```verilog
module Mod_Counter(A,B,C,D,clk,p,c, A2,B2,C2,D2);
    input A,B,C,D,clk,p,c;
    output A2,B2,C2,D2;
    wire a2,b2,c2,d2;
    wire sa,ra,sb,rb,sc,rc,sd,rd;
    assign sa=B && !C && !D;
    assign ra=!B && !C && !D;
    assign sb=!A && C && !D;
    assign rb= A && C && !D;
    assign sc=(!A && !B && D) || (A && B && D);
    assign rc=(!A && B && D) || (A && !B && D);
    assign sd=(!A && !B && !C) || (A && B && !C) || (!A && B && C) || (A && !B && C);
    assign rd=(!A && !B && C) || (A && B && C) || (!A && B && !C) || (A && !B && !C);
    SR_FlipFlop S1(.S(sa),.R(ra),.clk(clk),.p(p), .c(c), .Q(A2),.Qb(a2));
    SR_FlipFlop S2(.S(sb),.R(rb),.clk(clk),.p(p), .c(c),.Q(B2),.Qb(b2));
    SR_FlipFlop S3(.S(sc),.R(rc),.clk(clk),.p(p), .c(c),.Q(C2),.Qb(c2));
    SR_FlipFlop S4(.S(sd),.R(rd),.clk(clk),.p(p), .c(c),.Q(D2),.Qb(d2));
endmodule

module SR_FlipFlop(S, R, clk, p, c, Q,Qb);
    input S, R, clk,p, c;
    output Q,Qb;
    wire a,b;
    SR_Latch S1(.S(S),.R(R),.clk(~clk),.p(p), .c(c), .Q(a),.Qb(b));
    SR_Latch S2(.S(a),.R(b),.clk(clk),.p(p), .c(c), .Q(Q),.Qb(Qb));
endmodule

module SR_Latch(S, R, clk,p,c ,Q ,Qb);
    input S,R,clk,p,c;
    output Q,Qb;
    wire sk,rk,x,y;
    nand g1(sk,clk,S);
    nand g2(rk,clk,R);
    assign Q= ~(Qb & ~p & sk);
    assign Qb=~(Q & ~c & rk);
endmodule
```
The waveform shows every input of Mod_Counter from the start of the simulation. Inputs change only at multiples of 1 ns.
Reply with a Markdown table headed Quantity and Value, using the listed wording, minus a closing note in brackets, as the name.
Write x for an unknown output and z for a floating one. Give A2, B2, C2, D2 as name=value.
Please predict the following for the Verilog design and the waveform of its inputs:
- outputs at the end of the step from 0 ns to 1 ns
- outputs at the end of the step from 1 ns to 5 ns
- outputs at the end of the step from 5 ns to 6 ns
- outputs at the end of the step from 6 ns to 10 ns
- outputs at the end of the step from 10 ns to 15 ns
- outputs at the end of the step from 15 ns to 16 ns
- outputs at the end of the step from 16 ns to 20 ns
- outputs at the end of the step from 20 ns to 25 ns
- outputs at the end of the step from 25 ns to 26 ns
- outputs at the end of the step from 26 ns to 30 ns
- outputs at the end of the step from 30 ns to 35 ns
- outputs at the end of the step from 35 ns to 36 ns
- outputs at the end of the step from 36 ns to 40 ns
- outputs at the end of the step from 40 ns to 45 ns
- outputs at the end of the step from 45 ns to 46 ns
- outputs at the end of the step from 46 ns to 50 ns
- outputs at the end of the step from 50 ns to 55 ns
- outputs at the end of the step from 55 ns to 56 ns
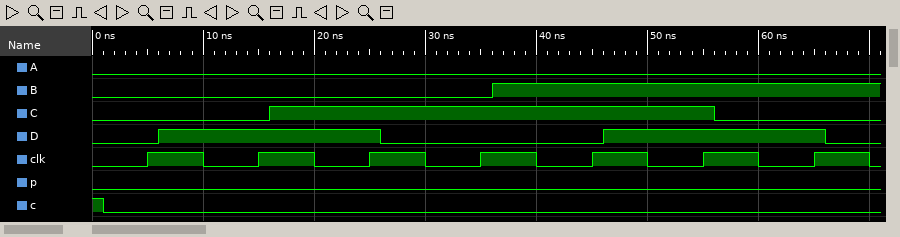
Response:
| Quantity | Value |
|---|---|
| outputs at the end of the step from 0 ns to 1 ns | A2=0, B2=0, C2=0, D2=0 |
| outputs at the end of the step from 1 ns to 5 ns | A2=0, B2=0, C2=0, D2=0 |
| outputs at the end of the step from 5 ns to 6 ns | A2=0, B2=0, C2=0, D2=1 |
| outputs at the end of the step from 6 ns to 10 ns | A2=0, B2=0, C2=0, D2=1 |
| outputs at the end of the step from 10 ns to 15 ns | A2=0, B2=0, C2=0, D2=1 |
| outputs at the end of the step from 15 ns to 16 ns | A2=0, B2=0, C2=1, D2=1 |
| outputs at the end of the step from 16 ns to 20 ns | A2=0, B2=0, C2=1, D2=1 |
| outputs at the end of the step from 20 ns to 25 ns | A2=0, B2=0, C2=1, D2=1 |
| outputs at the end of the step from 25 ns to 26 ns | A2=0, B2=0, C2=1, D2=0 |
| outputs at the end of the step from 26 ns to 30 ns | A2=0, B2=0, C2=1, D2=0 |
| outputs at the end of the step from 30 ns to 35 ns | A2=0, B2=0, C2=1, D2=0 |
| outputs at the end of the step from 35 ns to 36 ns | A2=0, B2=1, C2=1, D2=0 |
| outputs at the end of the step from 36 ns to 40 ns | A2=0, B2=1, C2=1, D2=0 |
| outputs at the end of the step from 40 ns to 45 ns | A2=0, B2=1, C2=1, D2=0 |
| outputs at the end of the step from 45 ns to 46 ns | A2=0, B2=1, C2=1, D2=1 |
| outputs at the end of the step from 46 ns to 50 ns | A2=0, B2=1, C2=1, D2=1 |
| outputs at the end of the step from 50 ns to 55 ns | A2=0, B2=1, C2=1, D2=1 |
| outputs at the end of the step from 55 ns to 56 ns | A2=0, B2=1, C2=0, D2=1 |
